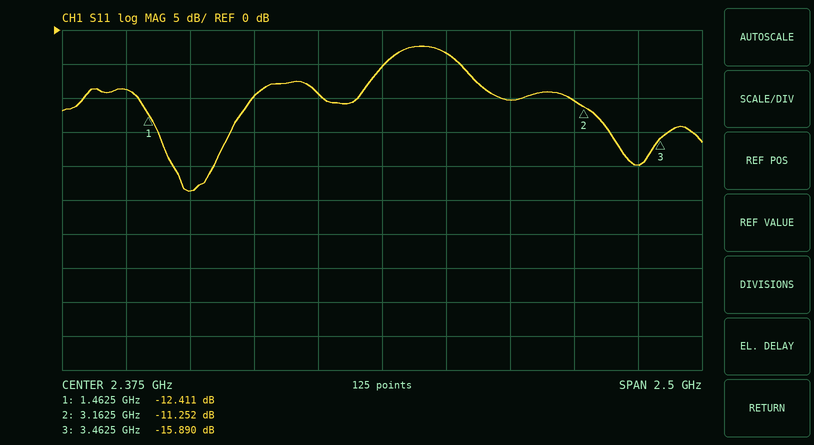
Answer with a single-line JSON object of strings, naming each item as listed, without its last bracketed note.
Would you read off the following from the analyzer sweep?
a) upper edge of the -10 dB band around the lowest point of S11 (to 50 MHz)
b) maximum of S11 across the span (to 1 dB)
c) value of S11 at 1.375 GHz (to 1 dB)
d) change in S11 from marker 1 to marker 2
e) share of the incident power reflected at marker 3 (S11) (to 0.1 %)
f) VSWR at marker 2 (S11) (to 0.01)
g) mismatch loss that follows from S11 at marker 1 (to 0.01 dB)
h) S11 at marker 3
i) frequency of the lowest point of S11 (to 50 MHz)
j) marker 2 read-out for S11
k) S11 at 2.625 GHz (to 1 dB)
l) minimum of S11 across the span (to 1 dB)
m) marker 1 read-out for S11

{"upper edge of the -10 dB band around the lowest point of S11": "1.85 GHz", "maximum of S11 across the span": "-2 dB", "value of S11 at 1.375 GHz": "-9 dB", "change in S11 from marker 1 to marker 2": "1.159 dB", "share of the incident power reflected at marker 3 (S11)": "2.6 %", "VSWR at marker 2 (S11)": "1.75", "mismatch loss that follows from S11 at marker 1": "0.26 dB", "S11 at marker 3": "-15.890 dB", "frequency of the lowest point of S11": "1.60 GHz", "marker 2 read-out for S11": "-11.252 dB", "S11 at 2.625 GHz": "-3 dB", "minimum of S11 across the span": "-24 dB", "marker 1 read-out for S11": "-12.411 dB"}
